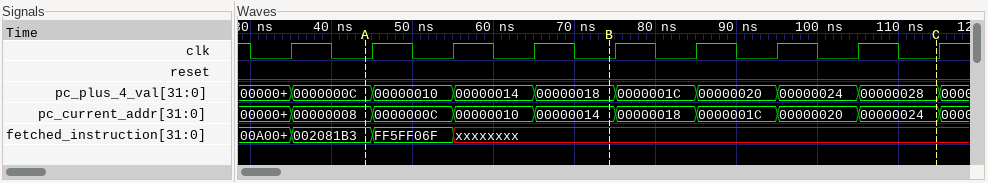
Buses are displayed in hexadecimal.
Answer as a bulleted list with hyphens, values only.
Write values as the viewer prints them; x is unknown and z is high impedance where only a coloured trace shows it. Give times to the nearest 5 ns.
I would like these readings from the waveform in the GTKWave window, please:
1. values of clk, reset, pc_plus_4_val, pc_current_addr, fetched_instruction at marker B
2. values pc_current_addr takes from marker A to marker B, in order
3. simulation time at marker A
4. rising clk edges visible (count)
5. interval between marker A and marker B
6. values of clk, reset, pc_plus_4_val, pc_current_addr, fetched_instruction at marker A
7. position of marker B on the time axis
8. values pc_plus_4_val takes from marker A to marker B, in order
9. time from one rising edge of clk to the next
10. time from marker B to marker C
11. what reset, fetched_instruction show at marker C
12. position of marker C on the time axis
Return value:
- clk=0, reset=0, pc_plus_4_val=00000018, pc_current_addr=00000014, fetched_instruction=xxxxxxxx
- 00000008, 0000000C, 00000010, 00000014
- 45 ns
- 9
- 30 ns
- clk=0, reset=0, pc_plus_4_val=0000000C, pc_current_addr=00000008, fetched_instruction=002081B3
- 75 ns
- 0000000C, 00000010, 00000014, 00000018
- 10 ns
- 40 ns
- reset=0, fetched_instruction=xxxxxxxx
- 115 ns
